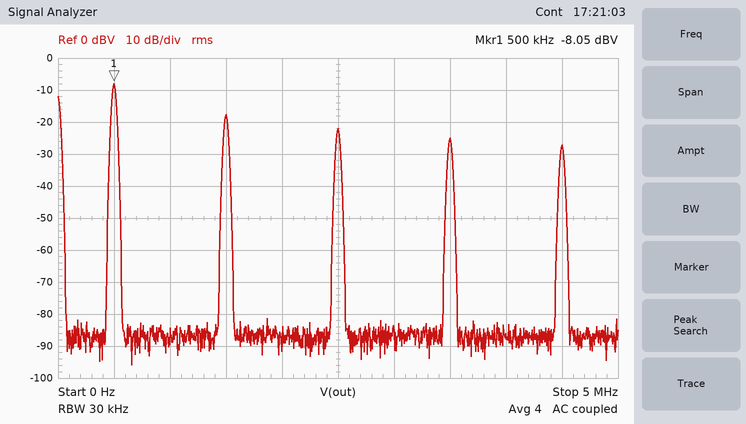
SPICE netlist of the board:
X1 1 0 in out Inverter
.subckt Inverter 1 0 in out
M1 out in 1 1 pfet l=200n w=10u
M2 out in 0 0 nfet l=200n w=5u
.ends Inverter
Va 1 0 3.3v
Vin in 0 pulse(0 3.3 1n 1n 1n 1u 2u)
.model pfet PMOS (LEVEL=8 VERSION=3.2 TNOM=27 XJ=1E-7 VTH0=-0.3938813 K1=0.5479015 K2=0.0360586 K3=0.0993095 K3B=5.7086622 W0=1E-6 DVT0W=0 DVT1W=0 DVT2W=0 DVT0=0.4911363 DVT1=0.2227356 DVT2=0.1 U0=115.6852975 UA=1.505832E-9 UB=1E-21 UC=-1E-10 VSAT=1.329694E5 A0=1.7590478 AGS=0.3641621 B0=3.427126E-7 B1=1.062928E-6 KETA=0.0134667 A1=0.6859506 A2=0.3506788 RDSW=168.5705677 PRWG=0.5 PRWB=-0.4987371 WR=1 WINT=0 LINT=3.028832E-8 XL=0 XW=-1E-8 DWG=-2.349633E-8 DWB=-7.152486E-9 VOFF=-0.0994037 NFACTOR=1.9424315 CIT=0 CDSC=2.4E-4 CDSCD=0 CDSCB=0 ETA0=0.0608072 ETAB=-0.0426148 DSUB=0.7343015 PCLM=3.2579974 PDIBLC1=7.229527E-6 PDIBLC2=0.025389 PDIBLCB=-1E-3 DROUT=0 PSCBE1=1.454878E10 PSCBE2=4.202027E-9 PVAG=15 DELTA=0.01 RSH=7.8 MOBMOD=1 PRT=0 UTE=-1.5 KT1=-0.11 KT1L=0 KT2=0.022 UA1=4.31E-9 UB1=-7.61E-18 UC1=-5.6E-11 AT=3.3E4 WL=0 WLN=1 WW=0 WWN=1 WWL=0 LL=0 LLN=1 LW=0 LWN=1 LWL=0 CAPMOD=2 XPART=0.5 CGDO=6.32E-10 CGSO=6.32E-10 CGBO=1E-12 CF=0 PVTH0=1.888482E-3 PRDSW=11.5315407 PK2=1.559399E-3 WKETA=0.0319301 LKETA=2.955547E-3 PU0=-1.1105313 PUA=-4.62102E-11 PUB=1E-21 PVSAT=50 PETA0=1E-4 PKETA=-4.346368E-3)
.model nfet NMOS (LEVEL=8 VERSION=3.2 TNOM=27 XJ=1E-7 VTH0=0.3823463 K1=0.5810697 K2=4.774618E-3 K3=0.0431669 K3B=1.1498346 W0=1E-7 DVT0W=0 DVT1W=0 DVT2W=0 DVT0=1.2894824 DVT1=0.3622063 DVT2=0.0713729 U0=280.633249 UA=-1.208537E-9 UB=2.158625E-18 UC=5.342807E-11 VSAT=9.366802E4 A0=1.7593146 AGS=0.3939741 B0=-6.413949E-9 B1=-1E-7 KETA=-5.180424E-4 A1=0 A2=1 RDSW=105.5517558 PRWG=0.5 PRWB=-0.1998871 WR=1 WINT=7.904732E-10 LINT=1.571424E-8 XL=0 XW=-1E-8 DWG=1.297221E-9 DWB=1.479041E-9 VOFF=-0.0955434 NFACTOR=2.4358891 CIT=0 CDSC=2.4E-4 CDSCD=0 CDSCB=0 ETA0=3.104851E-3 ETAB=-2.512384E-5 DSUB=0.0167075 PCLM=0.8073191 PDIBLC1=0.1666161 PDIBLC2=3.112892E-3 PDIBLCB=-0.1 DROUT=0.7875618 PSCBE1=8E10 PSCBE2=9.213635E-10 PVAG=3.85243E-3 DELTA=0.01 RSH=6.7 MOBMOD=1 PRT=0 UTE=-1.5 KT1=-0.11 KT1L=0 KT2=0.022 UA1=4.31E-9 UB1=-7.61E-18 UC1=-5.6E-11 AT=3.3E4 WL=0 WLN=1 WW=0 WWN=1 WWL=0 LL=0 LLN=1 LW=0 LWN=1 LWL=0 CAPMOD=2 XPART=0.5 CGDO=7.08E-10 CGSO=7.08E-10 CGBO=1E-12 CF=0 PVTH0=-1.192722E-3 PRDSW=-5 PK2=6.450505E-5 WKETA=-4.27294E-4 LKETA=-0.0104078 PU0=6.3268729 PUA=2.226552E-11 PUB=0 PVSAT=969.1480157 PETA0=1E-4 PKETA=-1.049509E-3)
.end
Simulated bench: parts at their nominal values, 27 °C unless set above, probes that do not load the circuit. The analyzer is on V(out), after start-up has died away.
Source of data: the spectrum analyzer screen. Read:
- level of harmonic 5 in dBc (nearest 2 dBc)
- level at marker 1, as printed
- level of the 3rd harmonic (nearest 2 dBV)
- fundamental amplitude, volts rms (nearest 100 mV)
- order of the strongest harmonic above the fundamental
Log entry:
-14 dBc
-8.05 dBV
-18 dBV
400 mV
3
